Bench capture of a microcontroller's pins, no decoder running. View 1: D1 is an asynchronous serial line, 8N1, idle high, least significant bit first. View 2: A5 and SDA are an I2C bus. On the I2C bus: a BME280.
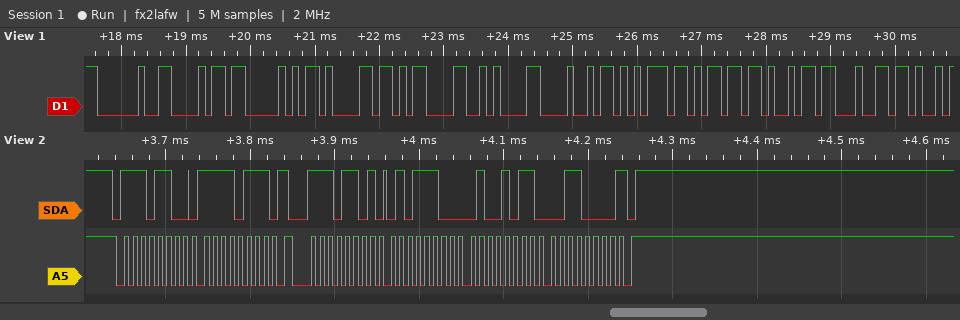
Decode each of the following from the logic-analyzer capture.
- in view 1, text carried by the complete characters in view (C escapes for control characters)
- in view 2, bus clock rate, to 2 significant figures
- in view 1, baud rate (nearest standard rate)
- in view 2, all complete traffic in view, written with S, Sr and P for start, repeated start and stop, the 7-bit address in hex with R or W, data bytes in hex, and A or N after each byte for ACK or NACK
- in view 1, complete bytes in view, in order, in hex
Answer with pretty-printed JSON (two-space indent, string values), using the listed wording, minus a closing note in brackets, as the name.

{
  "in view 1, text carried by the complete characters in view": "\" hPa\\r\\nHumid\"",
  "in view 2, bus clock rate, to 2 significant figures": "100 kHz",
  "in view 1, baud rate": "9600 baud",
  "in view 2, all complete traffic in view, written with S, Sr and P for start, repeated start and stop, the 7-bit address in hex with R or W, data bytes in hex, and A or N after each byte for ACK or NACK": "S 76W A F7 A Sr 76R A 5C A 4B A 30 N P",
  "in view 1, complete bytes in view, in order, in hex": "0x20 0x68 0x50 0x61 0x0D 0x0A 0x48 0x75 0x6D 0x69 0x64"
}
